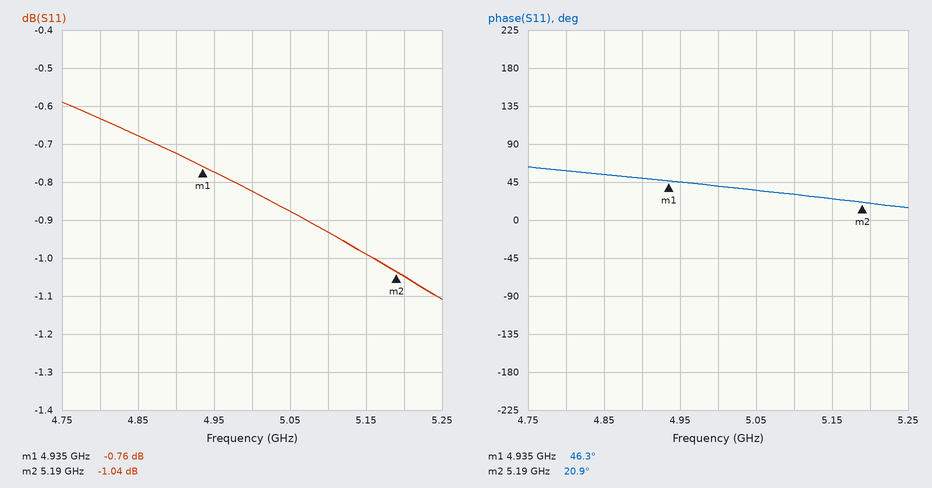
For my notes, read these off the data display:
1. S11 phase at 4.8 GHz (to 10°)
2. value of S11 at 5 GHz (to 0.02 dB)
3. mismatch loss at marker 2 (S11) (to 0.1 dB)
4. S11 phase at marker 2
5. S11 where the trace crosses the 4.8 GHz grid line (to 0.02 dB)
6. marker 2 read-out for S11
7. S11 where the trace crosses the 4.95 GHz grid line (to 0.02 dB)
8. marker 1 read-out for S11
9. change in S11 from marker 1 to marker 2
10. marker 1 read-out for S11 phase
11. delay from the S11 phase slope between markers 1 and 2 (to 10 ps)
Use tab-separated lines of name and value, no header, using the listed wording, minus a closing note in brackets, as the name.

S11 phase at 4.8 GHz	60°
value of S11 at 5 GHz	-0.82 dB
mismatch loss at marker 2 (S11)	6.7 dB
S11 phase at marker 2	20.9°
S11 where the trace crosses the 4.8 GHz grid line	-0.64 dB
marker 2 read-out for S11	-1.04 dB
S11 where the trace crosses the 4.95 GHz grid line	-0.78 dB
marker 1 read-out for S11	-0.76 dB
change in S11 from marker 1 to marker 2	-0.28 dB
marker 1 read-out for S11 phase	46.3°
delay from the S11 phase slope between markers 1 and 2	280 ps
